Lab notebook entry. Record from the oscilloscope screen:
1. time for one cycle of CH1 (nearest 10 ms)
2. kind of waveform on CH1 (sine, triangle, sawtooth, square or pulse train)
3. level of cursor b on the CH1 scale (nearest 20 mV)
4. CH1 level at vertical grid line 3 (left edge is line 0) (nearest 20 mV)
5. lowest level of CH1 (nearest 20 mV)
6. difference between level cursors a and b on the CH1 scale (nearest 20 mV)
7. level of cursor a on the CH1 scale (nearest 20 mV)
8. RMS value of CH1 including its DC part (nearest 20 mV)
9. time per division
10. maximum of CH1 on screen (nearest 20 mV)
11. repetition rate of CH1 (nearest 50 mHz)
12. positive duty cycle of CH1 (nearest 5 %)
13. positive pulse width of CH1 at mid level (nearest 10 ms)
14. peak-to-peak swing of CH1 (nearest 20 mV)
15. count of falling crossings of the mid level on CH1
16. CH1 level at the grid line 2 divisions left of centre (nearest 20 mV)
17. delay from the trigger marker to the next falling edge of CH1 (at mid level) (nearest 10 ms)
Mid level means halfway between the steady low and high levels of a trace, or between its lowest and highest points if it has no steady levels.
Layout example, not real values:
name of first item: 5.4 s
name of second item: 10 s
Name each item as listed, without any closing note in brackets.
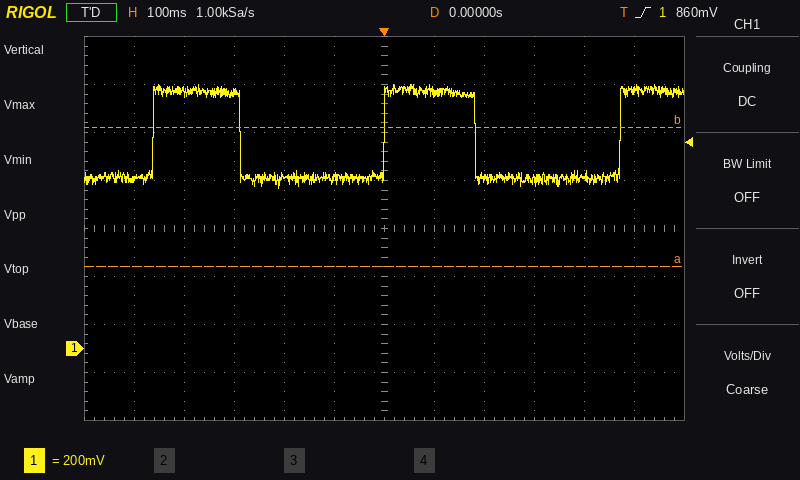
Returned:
time for one cycle of CH1: 470 ms
kind of waveform on CH1: pulse train
level of cursor b on the CH1 scale: 920 mV
CH1 level at vertical grid line 3 (left edge is line 0): 1.06 V
lowest level of CH1: 660 mV
difference between level cursors a and b on the CH1 scale: 580 mV
level of cursor a on the CH1 scale: 340 mV
RMS value of CH1 including its DC part: 860 mV
time per division: 100 ms
maximum of CH1 on screen: 1.10 V
repetition rate of CH1: 2.15 Hz
positive duty cycle of CH1: 40 %
positive pulse width of CH1 at mid level: 180 ms
peak-to-peak swing of CH1: 440 mV
count of falling crossings of the mid level on CH1: 2
CH1 level at the grid line 2 divisions left of centre: 720 mV
delay from the trigger marker to the next falling edge of CH1 (at mid level): 180 ms
